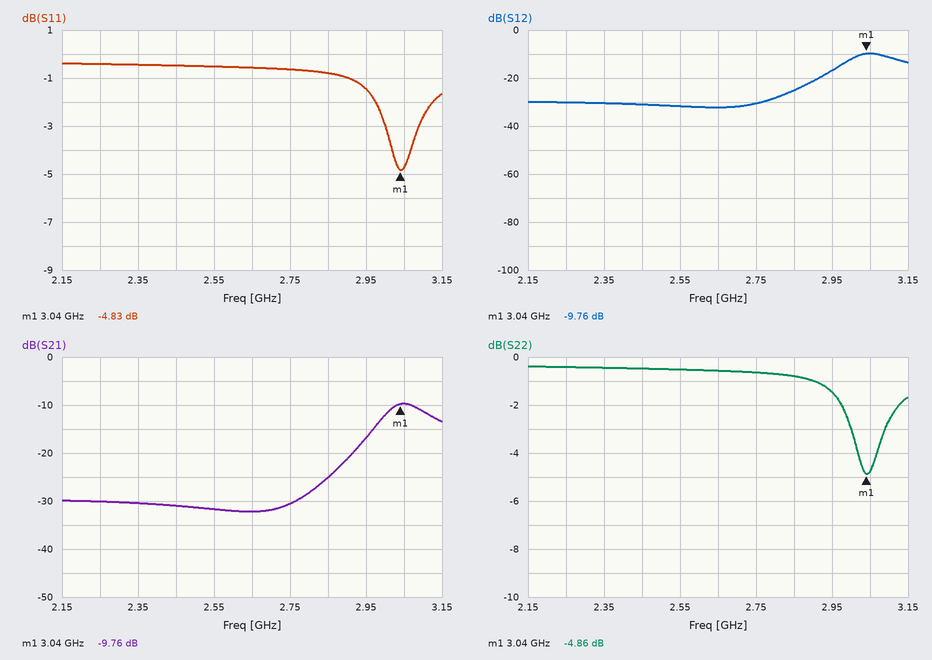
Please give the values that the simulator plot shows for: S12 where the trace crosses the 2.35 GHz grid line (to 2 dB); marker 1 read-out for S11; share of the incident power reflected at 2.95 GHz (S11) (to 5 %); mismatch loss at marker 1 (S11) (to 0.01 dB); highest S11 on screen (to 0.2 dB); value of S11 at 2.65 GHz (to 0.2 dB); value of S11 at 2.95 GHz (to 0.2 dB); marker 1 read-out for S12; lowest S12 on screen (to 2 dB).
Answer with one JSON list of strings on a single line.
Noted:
["-30 dB", "-4.83 dB", "70 %", "1.73 dB", "-0.4 dB", "-0.6 dB", "-1.4 dB", "-9.76 dB", "-32 dB"]
